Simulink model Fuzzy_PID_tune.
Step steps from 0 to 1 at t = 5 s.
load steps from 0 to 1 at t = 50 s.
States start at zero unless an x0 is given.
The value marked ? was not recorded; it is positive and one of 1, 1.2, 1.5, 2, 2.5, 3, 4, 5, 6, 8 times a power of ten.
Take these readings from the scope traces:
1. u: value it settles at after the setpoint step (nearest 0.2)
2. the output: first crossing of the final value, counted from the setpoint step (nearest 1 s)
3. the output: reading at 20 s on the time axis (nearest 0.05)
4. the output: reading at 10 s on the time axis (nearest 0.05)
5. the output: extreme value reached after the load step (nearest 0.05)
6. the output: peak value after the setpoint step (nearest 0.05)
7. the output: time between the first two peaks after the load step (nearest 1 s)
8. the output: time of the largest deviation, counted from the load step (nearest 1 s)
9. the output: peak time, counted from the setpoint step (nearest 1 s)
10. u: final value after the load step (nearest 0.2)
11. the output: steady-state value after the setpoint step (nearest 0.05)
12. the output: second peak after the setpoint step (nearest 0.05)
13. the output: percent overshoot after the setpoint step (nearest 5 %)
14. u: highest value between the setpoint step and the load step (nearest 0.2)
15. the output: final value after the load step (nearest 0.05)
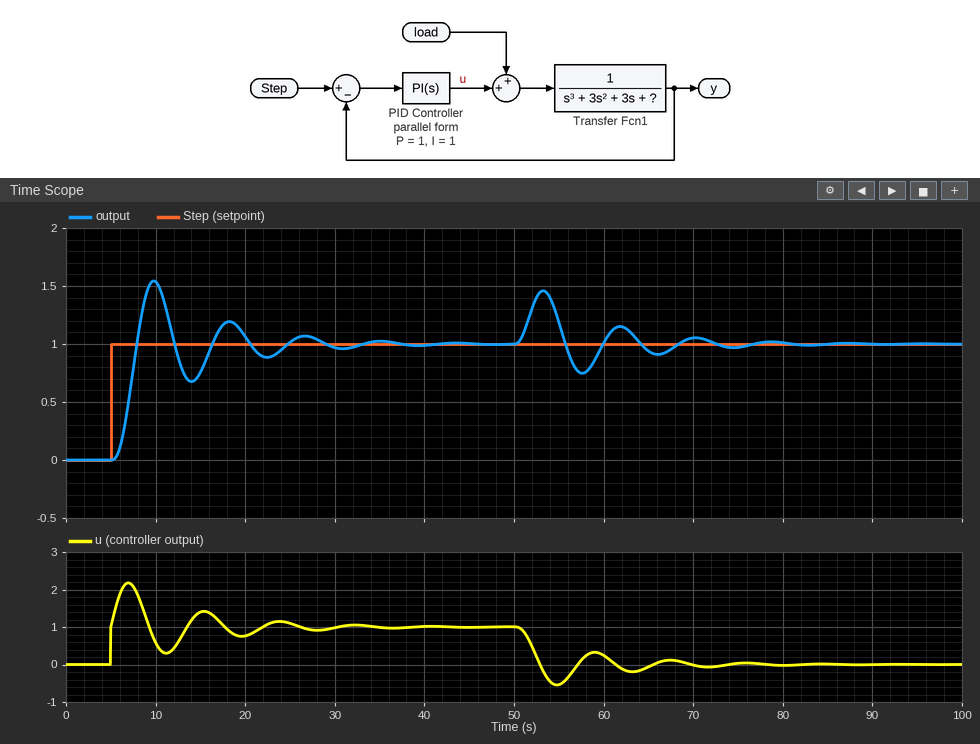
1.0
3 s
1.05
1.55
1.45
1.55
9 s
3 s
5 s
0.0
1.00
1.20
55 %
2.2
1.00
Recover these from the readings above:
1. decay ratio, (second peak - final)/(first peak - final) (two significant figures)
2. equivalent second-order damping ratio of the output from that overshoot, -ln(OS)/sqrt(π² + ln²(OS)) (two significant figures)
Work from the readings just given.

0.36
0.19
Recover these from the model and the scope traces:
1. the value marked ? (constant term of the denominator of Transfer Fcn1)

1
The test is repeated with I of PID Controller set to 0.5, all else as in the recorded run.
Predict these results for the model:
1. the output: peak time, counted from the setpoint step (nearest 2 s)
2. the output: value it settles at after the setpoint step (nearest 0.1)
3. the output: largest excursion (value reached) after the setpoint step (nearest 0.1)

6 s
1.0
1.1
